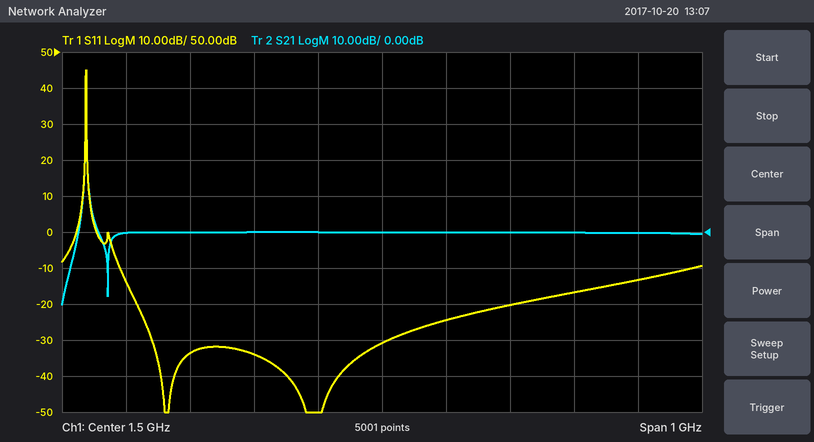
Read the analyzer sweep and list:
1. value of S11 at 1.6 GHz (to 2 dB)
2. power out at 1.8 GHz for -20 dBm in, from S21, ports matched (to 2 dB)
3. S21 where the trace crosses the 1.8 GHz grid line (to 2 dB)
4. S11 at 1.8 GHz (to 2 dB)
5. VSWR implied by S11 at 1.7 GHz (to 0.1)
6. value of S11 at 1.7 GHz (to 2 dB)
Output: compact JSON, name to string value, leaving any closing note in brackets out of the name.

{"value of S11 at 1.6 GHz": "-24 dB", "power out at 1.8 GHz for -20 dBm in, from S21, ports matched": "-20 dBm", "S21 where the trace crosses the 1.8 GHz grid line": "0 dB", "S11 at 1.8 GHz": "-16 dB", "VSWR implied by S11 at 1.7 GHz": "1.2", "value of S11 at 1.7 GHz": "-20 dB"}
